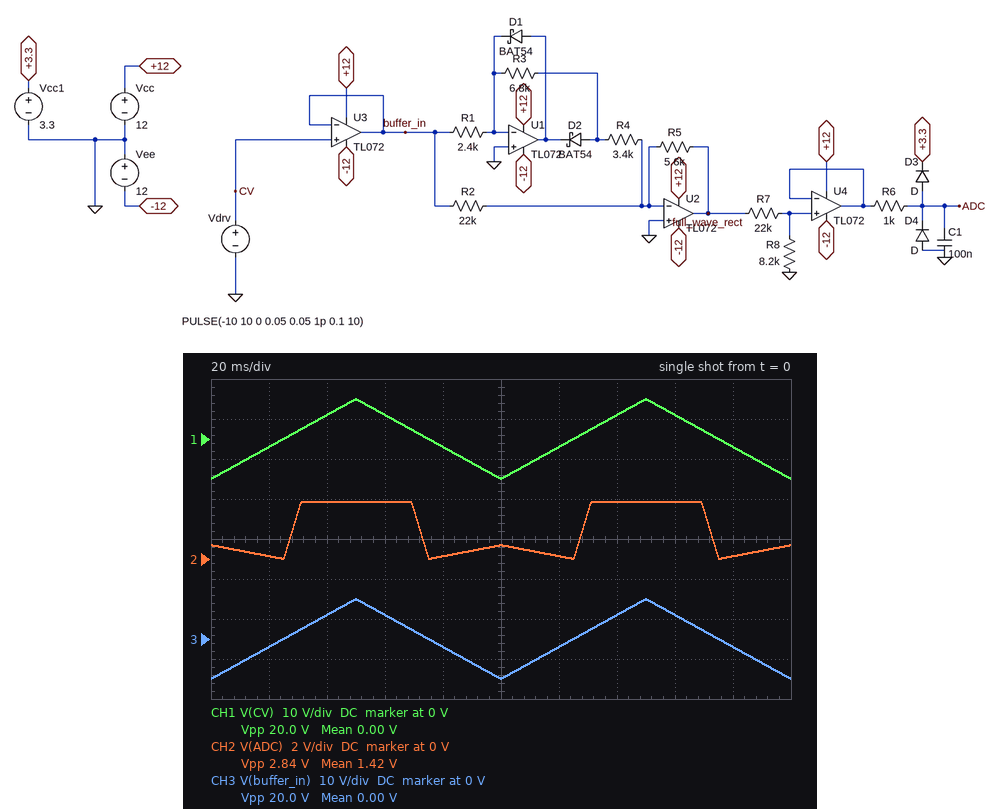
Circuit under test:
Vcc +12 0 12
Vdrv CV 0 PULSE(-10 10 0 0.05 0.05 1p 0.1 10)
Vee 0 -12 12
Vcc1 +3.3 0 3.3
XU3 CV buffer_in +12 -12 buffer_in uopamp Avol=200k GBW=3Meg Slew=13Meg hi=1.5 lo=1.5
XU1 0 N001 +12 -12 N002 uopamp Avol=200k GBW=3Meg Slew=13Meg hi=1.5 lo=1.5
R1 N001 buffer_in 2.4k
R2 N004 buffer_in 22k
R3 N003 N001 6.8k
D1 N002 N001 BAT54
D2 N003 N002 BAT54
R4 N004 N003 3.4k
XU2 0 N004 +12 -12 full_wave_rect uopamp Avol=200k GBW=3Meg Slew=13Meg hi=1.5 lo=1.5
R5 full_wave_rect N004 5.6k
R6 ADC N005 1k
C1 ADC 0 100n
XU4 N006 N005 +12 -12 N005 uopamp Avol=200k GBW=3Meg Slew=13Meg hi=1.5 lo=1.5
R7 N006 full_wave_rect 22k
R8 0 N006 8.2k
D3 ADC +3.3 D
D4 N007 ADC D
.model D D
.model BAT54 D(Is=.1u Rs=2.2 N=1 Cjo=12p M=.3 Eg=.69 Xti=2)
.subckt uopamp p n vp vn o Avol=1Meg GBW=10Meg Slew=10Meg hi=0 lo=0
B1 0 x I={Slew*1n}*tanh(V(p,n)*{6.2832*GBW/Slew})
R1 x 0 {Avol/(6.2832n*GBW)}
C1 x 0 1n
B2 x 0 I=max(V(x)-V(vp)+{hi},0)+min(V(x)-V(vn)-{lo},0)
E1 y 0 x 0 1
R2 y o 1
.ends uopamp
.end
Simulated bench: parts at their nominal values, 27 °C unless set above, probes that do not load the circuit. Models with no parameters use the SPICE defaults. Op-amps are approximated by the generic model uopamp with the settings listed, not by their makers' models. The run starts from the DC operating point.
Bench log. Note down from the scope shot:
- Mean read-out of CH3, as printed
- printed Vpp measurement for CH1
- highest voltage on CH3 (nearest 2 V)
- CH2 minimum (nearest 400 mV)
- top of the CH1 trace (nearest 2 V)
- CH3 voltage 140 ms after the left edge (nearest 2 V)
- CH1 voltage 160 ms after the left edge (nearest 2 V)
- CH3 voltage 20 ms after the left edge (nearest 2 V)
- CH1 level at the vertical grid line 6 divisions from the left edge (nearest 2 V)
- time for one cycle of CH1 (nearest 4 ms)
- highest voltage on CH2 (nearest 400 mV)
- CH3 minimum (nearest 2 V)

0.00 V
20.0 V
10 V
0 V
10 V
6 V
6 V
-2 V
-2 V
100 ms
2.8 V
-10 V
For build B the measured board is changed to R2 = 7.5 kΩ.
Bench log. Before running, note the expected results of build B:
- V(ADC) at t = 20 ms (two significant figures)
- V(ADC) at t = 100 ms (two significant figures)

410 mV
2.0 V
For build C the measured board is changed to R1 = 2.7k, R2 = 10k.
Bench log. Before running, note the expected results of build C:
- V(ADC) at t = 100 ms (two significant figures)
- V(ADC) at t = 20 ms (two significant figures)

1.5 V
310 mV
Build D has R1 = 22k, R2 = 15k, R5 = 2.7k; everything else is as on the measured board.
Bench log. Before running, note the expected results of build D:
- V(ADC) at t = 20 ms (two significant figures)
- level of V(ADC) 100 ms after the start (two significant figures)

100 mV
490 mV
